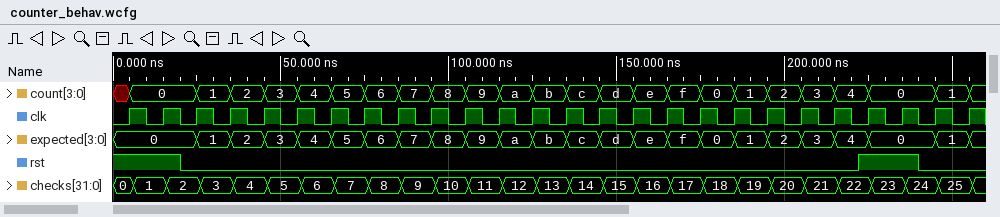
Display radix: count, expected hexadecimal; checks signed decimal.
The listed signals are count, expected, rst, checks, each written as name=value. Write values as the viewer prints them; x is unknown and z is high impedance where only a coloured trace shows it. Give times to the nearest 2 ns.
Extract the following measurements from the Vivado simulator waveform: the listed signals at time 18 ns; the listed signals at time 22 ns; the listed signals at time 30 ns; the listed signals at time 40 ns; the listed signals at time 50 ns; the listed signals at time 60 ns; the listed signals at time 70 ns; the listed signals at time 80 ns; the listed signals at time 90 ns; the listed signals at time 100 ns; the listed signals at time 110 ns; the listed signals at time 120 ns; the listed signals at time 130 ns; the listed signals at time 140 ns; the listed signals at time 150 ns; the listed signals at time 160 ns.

count=0, expected=0, rst=1, checks=2
count=0, expected=0, rst=0, checks=2
count=1, expected=1, rst=0, checks=3
count=2, expected=2, rst=0, checks=4
count=3, expected=3, rst=0, checks=5
count=4, expected=4, rst=0, checks=6
count=5, expected=5, rst=0, checks=7
count=6, expected=6, rst=0, checks=8
count=7, expected=7, rst=0, checks=9
count=8, expected=8, rst=0, checks=10
count=9, expected=9, rst=0, checks=11
count=a, expected=a, rst=0, checks=12
count=b, expected=b, rst=0, checks=13
count=c, expected=c, rst=0, checks=14
count=d, expected=d, rst=0, checks=15
count=e, expected=e, rst=0, checks=16
